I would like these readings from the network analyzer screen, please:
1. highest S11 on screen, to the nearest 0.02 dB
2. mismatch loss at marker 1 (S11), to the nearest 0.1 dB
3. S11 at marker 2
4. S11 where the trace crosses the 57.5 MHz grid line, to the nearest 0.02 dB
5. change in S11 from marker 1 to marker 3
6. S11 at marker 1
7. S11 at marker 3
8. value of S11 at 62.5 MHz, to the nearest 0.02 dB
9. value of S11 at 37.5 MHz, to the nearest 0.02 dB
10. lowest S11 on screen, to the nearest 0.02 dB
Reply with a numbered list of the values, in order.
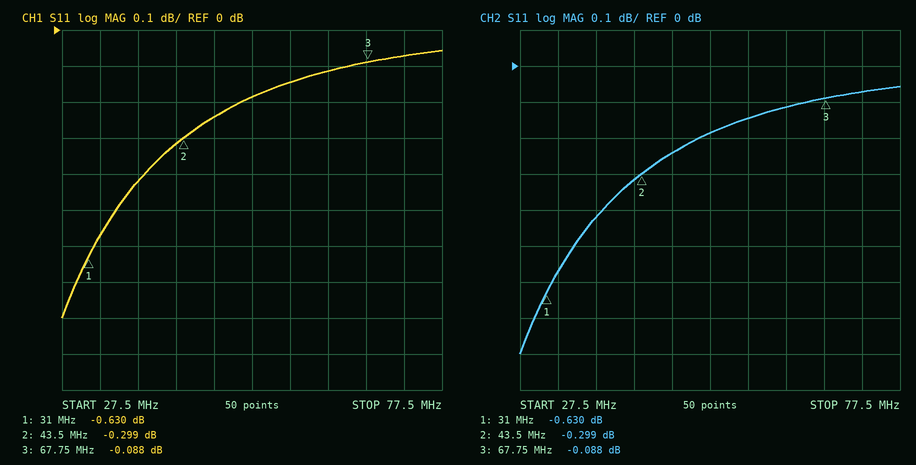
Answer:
1. -0.06 dB
2. 8.7 dB
3. -0.299 dB
4. -0.14 dB
5. 0.542 dB
6. -0.630 dB
7. -0.088 dB
8. -0.12 dB
9. -0.42 dB
10. -0.80 dB
